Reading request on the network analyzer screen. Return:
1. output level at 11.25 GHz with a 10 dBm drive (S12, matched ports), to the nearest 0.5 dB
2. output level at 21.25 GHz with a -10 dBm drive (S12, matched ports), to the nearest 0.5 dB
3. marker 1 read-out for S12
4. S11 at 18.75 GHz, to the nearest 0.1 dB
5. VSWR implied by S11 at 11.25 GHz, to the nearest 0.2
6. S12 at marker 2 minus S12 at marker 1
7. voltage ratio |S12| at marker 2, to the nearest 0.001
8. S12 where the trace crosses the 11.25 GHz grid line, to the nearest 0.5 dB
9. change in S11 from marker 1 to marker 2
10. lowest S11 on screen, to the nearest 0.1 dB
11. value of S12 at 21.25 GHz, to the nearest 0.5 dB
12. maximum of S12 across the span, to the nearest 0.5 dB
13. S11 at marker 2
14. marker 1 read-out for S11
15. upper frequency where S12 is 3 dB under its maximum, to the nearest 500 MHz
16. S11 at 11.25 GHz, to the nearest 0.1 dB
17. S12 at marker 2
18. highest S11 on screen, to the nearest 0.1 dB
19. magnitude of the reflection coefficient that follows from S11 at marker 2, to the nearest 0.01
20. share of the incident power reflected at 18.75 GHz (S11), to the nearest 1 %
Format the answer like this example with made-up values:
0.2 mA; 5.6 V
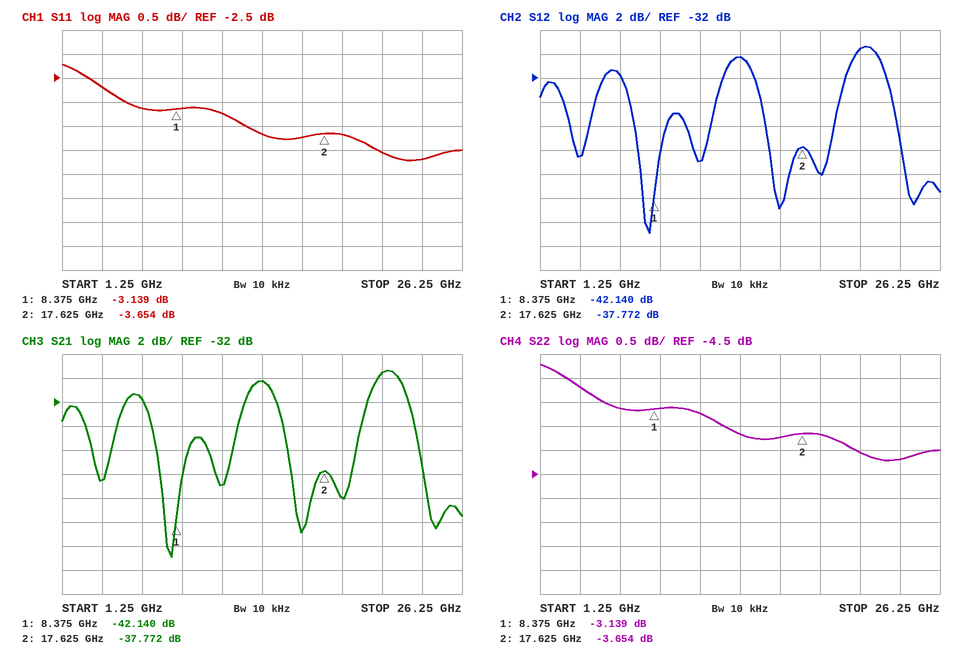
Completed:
-29.0 dBm; -39.5 dBm; -42.140 dB; -3.7 dB; 5.4; 4.368 dB; 0.013; -39.0 dB; -0.515 dB; -4.2 dB; -29.5 dB; -29.5 dB; -3.654 dB; -3.139 dB; 23.0 GHz; -3.2 dB; -37.772 dB; -2.2 dB; 0.66; 43 %
